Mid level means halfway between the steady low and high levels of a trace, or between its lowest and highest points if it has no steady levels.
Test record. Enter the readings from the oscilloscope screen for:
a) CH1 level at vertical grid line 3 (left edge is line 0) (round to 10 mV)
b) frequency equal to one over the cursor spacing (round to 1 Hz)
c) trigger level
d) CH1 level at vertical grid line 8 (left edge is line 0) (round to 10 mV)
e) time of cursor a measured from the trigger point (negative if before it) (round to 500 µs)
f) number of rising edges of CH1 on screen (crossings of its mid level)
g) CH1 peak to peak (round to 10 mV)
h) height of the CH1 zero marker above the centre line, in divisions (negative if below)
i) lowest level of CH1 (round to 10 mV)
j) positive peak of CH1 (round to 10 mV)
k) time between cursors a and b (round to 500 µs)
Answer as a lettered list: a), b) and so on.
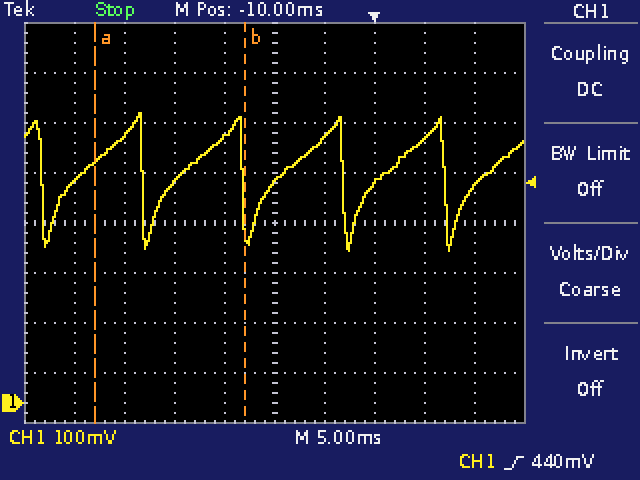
a) 440 mV
b) 67 Hz
c) 440 mV
d) 530 mV
e) -28.0 ms
f) 5
g) 280 mV
h) -3.6 div
i) 300 mV
j) 580 mV
k) 15.0 ms
